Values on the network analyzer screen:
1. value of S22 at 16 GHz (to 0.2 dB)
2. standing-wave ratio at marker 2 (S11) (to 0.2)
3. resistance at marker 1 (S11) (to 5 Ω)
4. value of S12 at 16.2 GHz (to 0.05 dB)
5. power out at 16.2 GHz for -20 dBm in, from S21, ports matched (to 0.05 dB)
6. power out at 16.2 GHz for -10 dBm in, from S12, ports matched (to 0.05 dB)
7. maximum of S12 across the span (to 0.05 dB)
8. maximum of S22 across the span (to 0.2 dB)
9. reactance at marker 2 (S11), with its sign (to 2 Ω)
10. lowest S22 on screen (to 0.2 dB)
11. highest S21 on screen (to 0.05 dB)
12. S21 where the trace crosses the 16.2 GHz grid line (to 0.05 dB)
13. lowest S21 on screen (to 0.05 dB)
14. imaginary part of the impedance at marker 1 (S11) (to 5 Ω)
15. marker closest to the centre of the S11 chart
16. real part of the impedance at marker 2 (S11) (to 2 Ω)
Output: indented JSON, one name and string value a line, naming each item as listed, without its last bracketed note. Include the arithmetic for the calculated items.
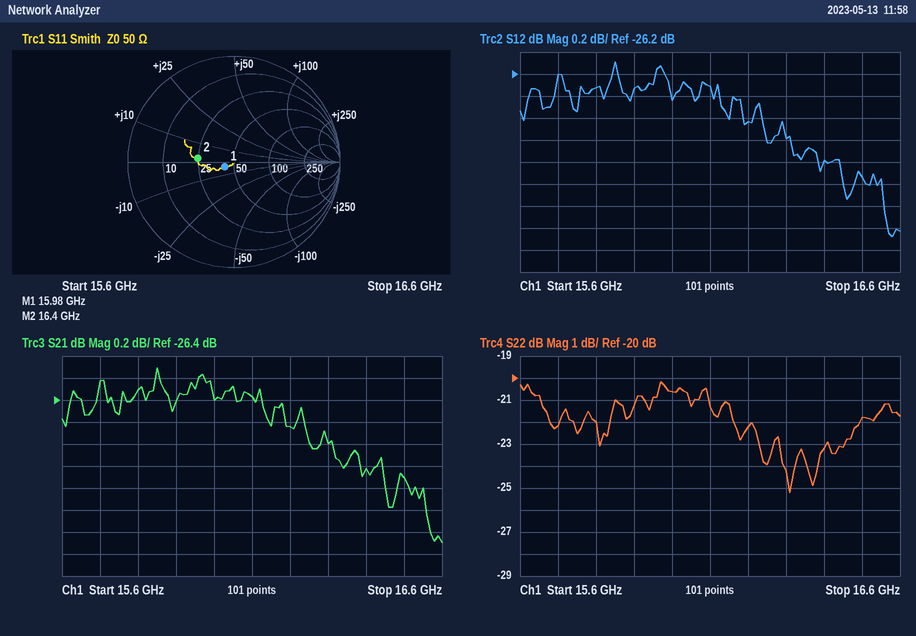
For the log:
{
  "value of S22 at 16 GHz": "-20.6 dB",
  "standing-wave ratio at marker 2 (S11)": "2.0",
  "resistance at marker 1 (S11)": "40 Ω",
  "value of S12 at 16.2 GHz": "-26.65 dB",
  "power out at 16.2 GHz for -20 dBm in, from S21, ports matched": "-20 dBm + (-26.65 dB) = -46.65 dBm",
  "power out at 16.2 GHz for -10 dBm in, from S12, ports matched": "-10 dBm + (-26.65 dB) = -36.65 dBm",
  "maximum of S12 across the span": "-26.10 dB",
  "maximum of S22 across the span": "-20.2 dB",
  "reactance at marker 2 (S11), with its sign": "+2 Ω",
  "lowest S22 on screen": "-25.2 dB",
  "highest S21 on screen": "-26.10 dB",
  "S21 where the trace crosses the 16.2 GHz grid line": "-26.65 dB",
  "lowest S21 on screen": "-27.70 dB",
  "imaginary part of the impedance at marker 1 (S11)": "-5 Ω",
  "marker closest to the centre of the S11 chart": "marker 1",
  "real part of the impedance at marker 2 (S11)": "24 Ω"
}
